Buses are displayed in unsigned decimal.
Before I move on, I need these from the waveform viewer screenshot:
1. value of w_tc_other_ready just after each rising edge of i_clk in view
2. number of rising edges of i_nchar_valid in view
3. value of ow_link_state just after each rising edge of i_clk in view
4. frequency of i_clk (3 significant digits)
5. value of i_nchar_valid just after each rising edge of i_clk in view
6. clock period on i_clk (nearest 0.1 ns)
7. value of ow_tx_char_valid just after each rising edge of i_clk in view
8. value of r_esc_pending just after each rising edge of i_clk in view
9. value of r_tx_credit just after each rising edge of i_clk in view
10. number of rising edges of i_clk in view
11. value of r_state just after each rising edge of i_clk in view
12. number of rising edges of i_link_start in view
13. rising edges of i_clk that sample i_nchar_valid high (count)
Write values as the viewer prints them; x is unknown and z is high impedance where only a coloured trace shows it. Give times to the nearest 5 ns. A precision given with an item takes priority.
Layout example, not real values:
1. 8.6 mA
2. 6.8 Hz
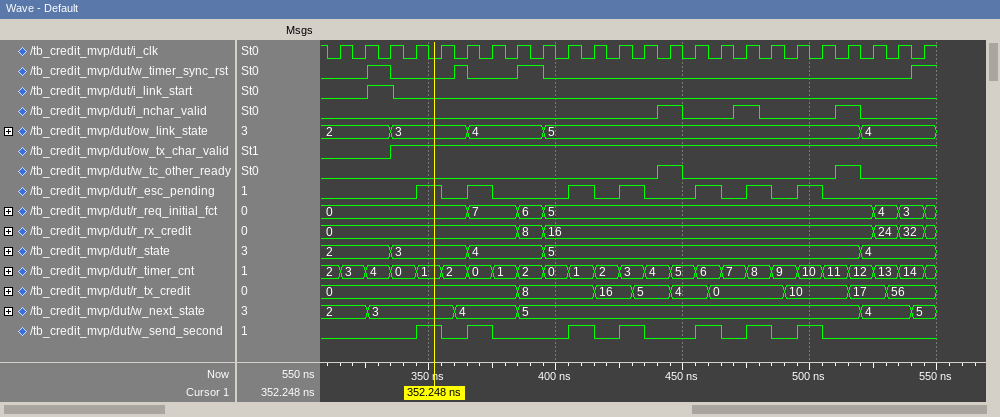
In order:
1. 0 0 0 0 0 0 0 0 0 0 0 0 0 1 0 0 0 0 0 0 1 0 0 0
2. 3
3. 2, 2, 3, 3, 3, 4, 4, 4, 5, 5, 5, 5, 5, 5, 5, 5, 5, 5, 5, 5, 5, 4, 4, 4
4. 100 MHz
5. 0 0 0 0 0 0 0 0 0 0 0 0 0 1 0 0 1 0 0 0 1 0 0 0
6. 10 ns
7. 0 0 1 1 1 1 1 1 1 1 1 1 1 1 1 1 1 1 1 1 1 1 1 1
8. 0 0 0 1 0 1 0 0 0 1 0 1 0 0 1 0 1 0 1 0 0 0 0 0
9. 0, 0, 0, 0, 0, 0, 0, 8, 8, 8, 16, 16, 5, 4, 4, 0, 0, 0, 10, 10, 17, 17, 56, 56
10. 24
11. 2, 2, 3, 3, 3, 4, 4, 4, 5, 5, 5, 5, 5, 5, 5, 5, 5, 5, 5, 5, 5, 4, 4, 4
12. 1
13. 3
